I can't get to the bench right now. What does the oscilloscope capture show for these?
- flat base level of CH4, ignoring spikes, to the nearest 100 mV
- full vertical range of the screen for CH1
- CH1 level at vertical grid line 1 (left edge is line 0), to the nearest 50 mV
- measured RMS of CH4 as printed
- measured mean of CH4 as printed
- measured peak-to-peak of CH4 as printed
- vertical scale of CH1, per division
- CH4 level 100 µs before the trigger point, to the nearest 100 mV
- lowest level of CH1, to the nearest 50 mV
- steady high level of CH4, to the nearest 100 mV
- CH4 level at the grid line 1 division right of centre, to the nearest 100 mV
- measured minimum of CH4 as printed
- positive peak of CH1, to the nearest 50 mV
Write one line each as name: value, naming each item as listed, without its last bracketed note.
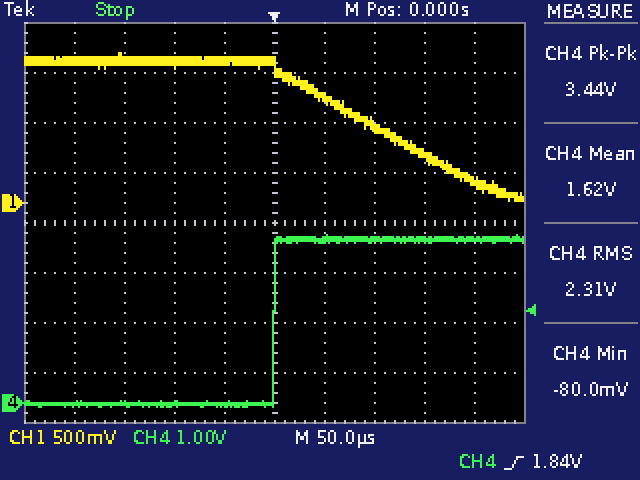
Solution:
flat base level of CH4, ignoring spikes, to the nearest 100 mV: 0.0 V
full vertical range of the screen for CH1: 4 V
CH1 level at vertical grid line 1 (left edge is line 0), to the nearest 50 mV: 1.40 V
measured RMS of CH4 as printed: 2.31 V
measured mean of CH4 as printed: 1.62 V
measured peak-to-peak of CH4 as printed: 3.44 V
vertical scale of CH1, per division: 500 mV
CH4 level 100 µs before the trigger point, to the nearest 100 mV: 0.0 V
lowest level of CH1, to the nearest 50 mV: 0 mV
steady high level of CH4, to the nearest 100 mV: 3.3 V
CH4 level at the grid line 1 division right of centre, to the nearest 100 mV: 3.3 V
measured minimum of CH4 as printed: -80.0 mV
positive peak of CH1, to the nearest 50 mV: 1.50 V
